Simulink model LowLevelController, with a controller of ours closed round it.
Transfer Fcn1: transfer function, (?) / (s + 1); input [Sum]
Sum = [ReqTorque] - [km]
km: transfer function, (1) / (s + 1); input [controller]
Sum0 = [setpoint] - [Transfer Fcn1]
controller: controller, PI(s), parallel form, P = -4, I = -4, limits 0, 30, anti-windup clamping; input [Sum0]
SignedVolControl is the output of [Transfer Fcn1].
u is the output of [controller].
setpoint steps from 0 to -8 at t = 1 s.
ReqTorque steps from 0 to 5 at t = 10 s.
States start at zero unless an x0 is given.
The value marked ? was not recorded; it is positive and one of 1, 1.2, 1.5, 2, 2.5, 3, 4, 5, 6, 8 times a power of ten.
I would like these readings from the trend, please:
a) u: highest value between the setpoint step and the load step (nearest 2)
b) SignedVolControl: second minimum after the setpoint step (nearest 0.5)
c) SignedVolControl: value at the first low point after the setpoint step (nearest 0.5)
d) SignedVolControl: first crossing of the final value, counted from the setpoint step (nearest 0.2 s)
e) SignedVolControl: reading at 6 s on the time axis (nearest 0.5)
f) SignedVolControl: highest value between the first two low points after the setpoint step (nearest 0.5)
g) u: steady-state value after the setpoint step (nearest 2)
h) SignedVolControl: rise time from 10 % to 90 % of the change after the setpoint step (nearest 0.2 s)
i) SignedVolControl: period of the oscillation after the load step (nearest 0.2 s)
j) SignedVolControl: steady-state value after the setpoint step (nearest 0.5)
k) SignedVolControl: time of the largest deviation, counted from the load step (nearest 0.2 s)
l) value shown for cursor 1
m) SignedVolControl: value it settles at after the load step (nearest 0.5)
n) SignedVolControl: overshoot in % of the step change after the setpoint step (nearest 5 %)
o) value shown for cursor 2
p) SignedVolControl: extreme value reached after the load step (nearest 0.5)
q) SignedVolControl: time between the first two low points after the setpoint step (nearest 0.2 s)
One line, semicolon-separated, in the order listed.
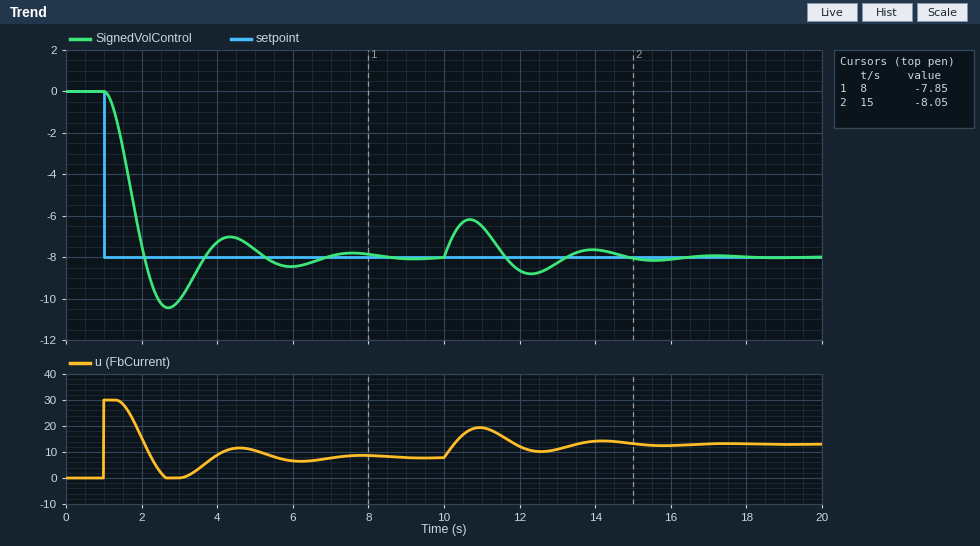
30; -8.5; -10.5; 1.0 s; -8.5; -7.0; 8; 0.8 s; 3.2 s; -8.0; 0.6 s; -7.85; -8.0; 30 %; -8.05; -6.0; 3.2 s
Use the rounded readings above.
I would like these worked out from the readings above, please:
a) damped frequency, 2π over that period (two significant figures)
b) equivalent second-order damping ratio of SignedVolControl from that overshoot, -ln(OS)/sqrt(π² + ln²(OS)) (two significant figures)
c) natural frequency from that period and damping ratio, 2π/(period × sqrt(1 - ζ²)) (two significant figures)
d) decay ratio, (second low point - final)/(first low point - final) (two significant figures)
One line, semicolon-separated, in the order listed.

2.0 rad/s; 0.36; 2.1 rad/s; 0.20
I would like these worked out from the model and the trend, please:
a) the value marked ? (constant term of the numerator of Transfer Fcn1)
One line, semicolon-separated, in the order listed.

1
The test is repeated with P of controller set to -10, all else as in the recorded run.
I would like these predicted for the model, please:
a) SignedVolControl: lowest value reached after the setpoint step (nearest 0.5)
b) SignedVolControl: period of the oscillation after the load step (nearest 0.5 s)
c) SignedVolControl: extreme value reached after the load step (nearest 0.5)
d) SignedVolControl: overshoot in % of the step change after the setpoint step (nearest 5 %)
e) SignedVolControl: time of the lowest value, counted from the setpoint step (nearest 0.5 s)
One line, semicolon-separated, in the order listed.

-9.5; 2.0 s; -6.5; 20 %; 1.5 s
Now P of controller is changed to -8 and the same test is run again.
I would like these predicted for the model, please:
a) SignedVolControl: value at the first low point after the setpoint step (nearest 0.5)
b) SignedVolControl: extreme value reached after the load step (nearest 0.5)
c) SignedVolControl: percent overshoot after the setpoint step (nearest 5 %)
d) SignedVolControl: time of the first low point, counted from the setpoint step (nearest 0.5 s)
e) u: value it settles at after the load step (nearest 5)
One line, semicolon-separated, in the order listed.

-9.5; -6.5; 15 %; 1.5 s; 15
